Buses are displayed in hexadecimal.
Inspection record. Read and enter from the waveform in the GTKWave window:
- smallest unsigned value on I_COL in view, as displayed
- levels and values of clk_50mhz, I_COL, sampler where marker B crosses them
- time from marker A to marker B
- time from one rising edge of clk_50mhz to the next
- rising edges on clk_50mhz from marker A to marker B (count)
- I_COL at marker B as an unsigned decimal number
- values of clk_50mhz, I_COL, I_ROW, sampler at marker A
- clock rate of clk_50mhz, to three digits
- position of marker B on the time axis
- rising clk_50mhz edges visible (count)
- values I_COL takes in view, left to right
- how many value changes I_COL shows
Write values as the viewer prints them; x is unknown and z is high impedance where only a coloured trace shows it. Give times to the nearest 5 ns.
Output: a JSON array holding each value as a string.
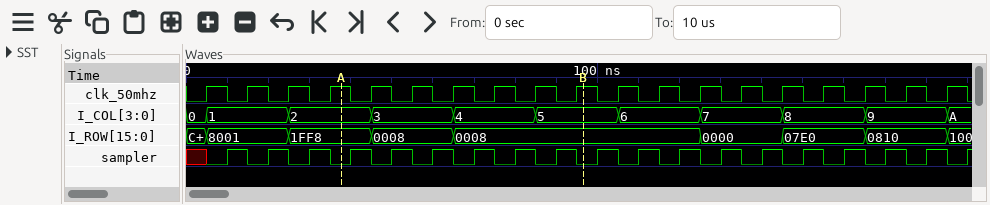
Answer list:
["0", "clk_50mhz=1, I_COL=5, sampler=0", "60 ns", "10 ns", "6", "5", "clk_50mhz=1, I_COL=2, I_ROW=1FF8, sampler=0", "100 MHz", "95 ns", "19", "0, 1, 2, 3, 4, 5, 6, 7, 8, 9, A", "10"]
